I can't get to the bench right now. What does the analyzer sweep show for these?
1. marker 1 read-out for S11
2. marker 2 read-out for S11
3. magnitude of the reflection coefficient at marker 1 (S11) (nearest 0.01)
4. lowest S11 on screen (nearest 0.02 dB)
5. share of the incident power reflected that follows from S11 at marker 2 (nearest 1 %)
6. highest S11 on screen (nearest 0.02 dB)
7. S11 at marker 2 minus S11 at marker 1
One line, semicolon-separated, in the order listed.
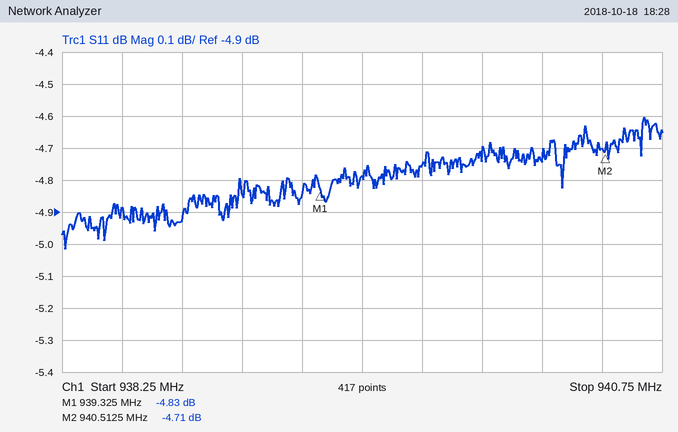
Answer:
-4.83 dB; -4.71 dB; 0.57; -5.02 dB; 34 %; -4.60 dB; 0.12 dB
